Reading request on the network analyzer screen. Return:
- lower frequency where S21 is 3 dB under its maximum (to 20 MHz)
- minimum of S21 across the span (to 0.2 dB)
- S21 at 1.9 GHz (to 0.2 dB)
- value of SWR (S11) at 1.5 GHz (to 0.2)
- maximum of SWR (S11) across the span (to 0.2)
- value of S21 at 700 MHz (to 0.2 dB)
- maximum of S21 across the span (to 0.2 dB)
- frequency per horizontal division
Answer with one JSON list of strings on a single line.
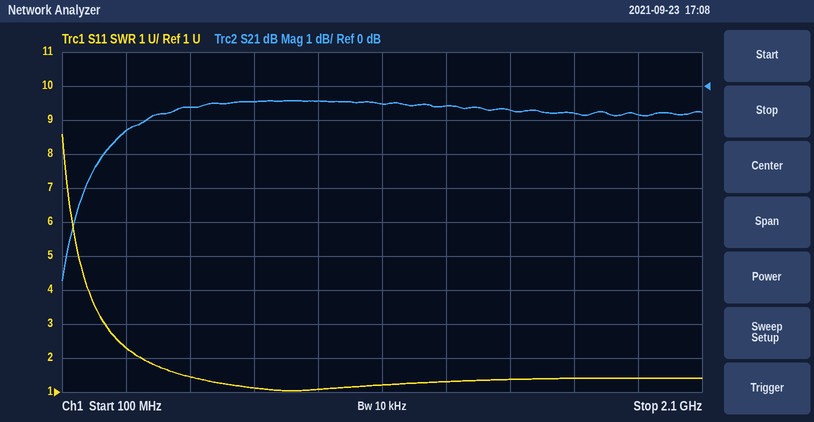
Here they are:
["160 MHz", "-5.8 dB", "-0.8 dB", "1.4", "8.6", "-0.4 dB", "-0.4 dB", "200 MHz"]
